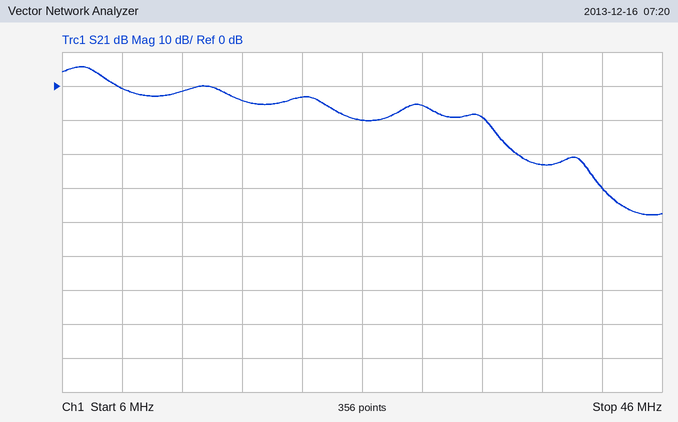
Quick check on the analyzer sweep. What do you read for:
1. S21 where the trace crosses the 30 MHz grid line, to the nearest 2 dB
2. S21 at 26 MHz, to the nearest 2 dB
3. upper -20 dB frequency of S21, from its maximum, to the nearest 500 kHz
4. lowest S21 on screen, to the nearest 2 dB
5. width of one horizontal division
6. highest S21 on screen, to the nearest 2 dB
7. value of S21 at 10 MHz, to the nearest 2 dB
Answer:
-6 dB
-10 dB
35.0 MHz
-38 dB
4 MHz
6 dB
0 dB
